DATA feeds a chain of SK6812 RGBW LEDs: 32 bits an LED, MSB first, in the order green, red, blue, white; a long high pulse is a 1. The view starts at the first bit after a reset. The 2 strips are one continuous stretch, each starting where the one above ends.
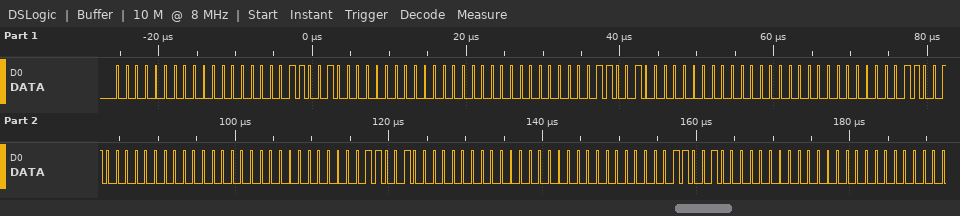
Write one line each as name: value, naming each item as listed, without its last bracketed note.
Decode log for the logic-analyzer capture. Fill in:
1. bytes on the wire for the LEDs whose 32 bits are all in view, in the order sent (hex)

bytes on the wire for the LEDs whose 32 bits are all in view, in the order sent: 00 00 32 00 00 00 32 00 00 00 32 00 00 00 32 00 00 00 32 00
